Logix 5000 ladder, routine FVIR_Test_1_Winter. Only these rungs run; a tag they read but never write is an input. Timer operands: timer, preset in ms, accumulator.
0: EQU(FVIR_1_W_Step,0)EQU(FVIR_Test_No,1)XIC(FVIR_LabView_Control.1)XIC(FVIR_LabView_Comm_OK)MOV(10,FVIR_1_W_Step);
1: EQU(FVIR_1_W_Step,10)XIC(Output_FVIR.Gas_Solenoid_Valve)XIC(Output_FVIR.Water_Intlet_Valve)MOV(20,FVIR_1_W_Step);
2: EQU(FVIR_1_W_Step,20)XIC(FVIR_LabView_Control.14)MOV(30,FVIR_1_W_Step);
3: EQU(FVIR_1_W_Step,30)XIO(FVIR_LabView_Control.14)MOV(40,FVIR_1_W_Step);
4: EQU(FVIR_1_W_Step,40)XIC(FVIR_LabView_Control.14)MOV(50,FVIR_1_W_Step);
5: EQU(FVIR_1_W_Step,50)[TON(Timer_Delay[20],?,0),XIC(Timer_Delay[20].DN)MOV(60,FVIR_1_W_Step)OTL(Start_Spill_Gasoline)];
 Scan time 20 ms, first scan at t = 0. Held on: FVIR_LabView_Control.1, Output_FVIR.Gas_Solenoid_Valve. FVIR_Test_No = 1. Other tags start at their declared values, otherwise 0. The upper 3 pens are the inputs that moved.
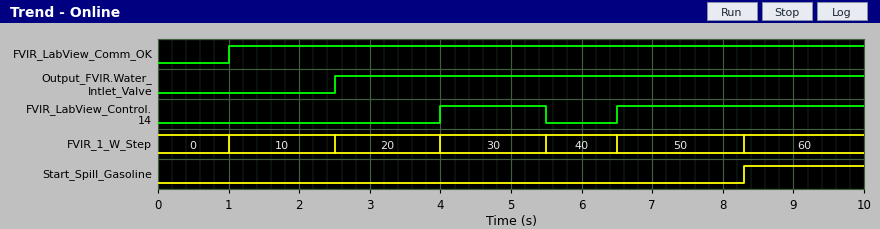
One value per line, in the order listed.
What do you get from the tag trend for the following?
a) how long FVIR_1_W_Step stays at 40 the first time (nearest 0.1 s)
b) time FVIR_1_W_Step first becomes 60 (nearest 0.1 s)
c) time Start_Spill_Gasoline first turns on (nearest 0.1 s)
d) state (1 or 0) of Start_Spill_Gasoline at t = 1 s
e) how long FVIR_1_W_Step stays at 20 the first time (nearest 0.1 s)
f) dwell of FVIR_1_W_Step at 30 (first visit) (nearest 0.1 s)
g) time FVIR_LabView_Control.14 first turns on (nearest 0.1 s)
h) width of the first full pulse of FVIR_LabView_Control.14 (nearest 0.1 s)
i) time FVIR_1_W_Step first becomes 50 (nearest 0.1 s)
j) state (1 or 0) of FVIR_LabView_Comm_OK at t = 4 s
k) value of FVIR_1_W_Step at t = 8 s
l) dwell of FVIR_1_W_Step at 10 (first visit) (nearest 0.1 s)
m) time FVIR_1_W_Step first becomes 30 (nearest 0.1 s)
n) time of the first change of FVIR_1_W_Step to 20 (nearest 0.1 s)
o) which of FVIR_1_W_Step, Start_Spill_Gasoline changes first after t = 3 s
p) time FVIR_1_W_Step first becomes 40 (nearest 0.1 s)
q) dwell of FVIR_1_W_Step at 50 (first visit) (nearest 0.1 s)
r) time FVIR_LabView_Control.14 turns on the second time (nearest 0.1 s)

1.0 s
8.3 s
8.3 s
0
1.5 s
1.5 s
4.0 s
1.5 s
6.5 s
1
50
1.5 s
4.0 s
2.5 s
FVIR_1_W_Step
5.5 s
1.8 s
6.5 s
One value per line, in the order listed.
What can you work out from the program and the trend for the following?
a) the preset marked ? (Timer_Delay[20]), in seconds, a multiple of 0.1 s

1.8 s
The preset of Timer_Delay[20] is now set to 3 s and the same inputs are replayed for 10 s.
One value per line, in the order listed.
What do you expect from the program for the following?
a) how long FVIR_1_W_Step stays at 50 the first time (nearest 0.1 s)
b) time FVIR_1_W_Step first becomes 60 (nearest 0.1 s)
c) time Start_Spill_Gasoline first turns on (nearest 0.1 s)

3.0 s
9.5 s
9.5 s
